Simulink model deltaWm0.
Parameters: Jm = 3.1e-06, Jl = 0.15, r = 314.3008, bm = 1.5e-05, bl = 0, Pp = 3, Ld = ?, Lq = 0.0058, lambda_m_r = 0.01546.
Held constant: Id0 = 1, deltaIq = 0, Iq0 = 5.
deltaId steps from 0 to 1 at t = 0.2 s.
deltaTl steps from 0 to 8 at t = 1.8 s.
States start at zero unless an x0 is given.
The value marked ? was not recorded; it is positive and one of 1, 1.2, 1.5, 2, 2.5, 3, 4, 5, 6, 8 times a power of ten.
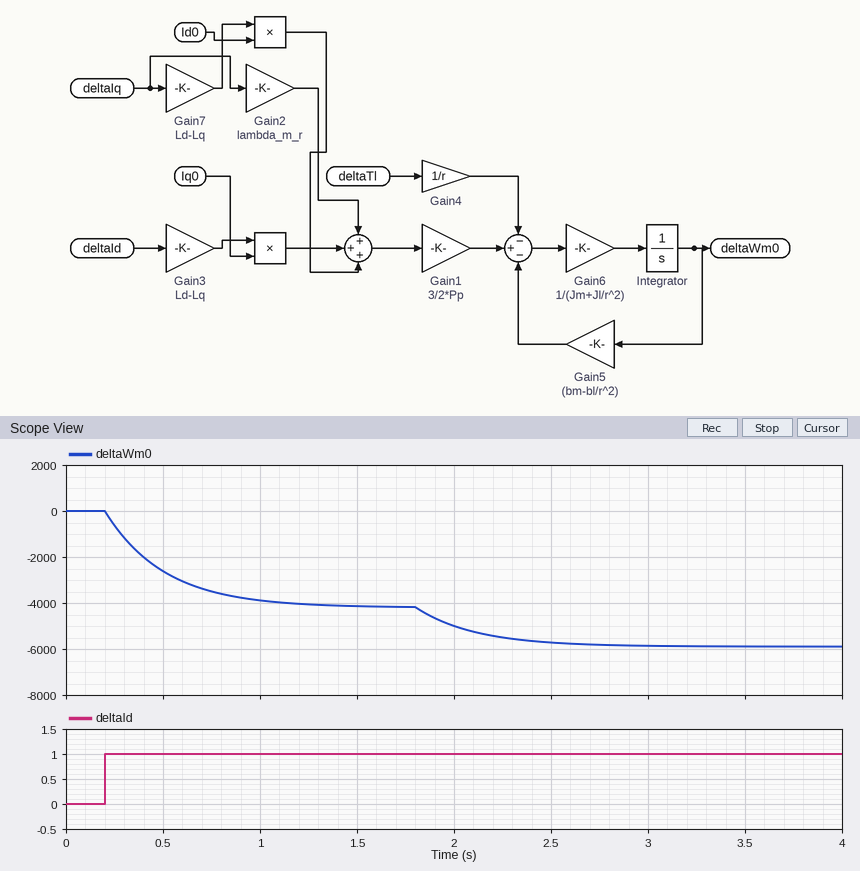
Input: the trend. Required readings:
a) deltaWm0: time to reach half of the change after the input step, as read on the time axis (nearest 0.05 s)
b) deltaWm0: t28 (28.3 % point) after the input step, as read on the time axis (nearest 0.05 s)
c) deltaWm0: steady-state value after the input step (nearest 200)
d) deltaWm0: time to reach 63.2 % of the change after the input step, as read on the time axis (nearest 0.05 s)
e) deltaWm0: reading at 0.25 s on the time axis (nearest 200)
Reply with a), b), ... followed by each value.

a) 0.40 s
b) 0.30 s
c) -4200
d) 0.50 s
e) -600
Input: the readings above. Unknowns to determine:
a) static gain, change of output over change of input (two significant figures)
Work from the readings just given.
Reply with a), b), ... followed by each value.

a) -4200
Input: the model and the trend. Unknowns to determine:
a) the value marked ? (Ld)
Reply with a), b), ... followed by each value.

a) 0.003
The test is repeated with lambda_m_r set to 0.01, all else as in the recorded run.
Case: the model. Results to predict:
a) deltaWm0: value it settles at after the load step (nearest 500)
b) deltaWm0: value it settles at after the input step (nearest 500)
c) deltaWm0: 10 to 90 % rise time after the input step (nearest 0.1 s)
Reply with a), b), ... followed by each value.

a) -6000
b) -4000
c) 0.7 s
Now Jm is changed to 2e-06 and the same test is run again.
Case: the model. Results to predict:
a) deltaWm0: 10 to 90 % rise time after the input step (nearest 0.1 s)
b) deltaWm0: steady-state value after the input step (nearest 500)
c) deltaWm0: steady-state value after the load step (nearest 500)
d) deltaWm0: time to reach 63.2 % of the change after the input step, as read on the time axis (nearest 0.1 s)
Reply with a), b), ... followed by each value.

a) 0.5 s
b) -4000
c) -6000
d) 0.4 s
